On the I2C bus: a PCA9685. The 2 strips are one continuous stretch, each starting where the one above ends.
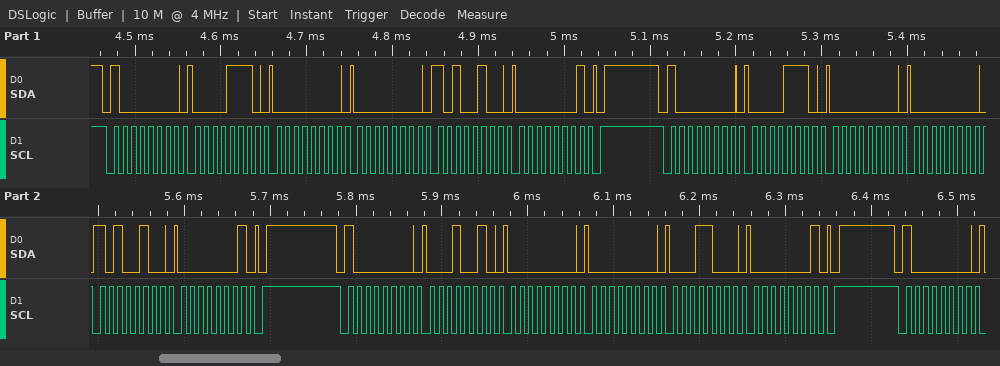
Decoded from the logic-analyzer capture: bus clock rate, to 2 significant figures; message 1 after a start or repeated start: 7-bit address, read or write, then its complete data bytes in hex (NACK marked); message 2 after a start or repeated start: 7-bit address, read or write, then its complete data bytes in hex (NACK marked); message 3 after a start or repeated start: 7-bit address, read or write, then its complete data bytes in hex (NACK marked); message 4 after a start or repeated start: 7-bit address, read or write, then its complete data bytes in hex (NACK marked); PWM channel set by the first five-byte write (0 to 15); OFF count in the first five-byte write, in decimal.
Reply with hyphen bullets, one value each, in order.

- 100 kHz
- 0x40 write: 0E 00 00 A4 01
- 0x40 write: 0E 00 00 A4 01
- 0x40 write: 12 00 00 18 01
- 0x40 write
- 2
- 420
